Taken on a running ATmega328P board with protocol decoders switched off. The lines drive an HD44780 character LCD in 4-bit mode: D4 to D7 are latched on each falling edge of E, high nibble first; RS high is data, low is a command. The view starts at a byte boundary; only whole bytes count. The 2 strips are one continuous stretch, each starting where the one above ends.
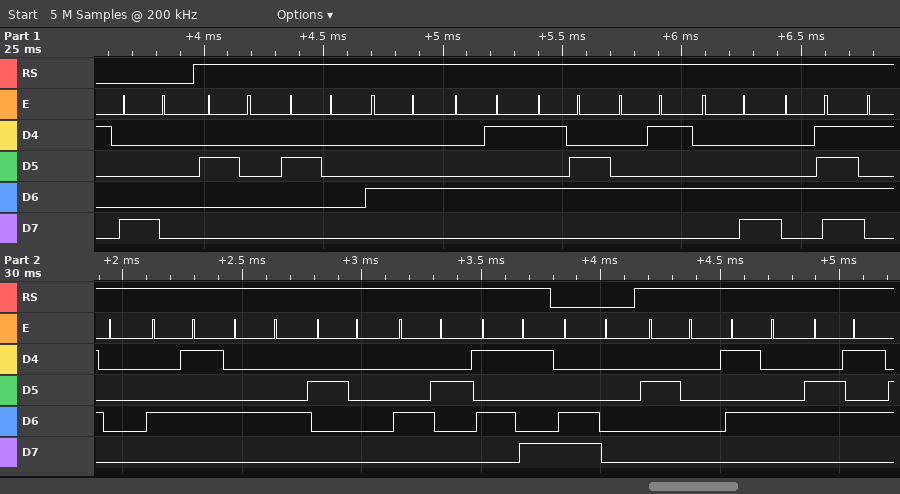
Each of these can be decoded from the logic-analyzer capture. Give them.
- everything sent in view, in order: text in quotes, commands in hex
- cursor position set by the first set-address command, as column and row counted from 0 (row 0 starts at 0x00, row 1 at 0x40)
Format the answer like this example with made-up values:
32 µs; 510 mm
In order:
0x80 "  DEVELOPED BY" 0xC0 " Te"; column 0, row 0
